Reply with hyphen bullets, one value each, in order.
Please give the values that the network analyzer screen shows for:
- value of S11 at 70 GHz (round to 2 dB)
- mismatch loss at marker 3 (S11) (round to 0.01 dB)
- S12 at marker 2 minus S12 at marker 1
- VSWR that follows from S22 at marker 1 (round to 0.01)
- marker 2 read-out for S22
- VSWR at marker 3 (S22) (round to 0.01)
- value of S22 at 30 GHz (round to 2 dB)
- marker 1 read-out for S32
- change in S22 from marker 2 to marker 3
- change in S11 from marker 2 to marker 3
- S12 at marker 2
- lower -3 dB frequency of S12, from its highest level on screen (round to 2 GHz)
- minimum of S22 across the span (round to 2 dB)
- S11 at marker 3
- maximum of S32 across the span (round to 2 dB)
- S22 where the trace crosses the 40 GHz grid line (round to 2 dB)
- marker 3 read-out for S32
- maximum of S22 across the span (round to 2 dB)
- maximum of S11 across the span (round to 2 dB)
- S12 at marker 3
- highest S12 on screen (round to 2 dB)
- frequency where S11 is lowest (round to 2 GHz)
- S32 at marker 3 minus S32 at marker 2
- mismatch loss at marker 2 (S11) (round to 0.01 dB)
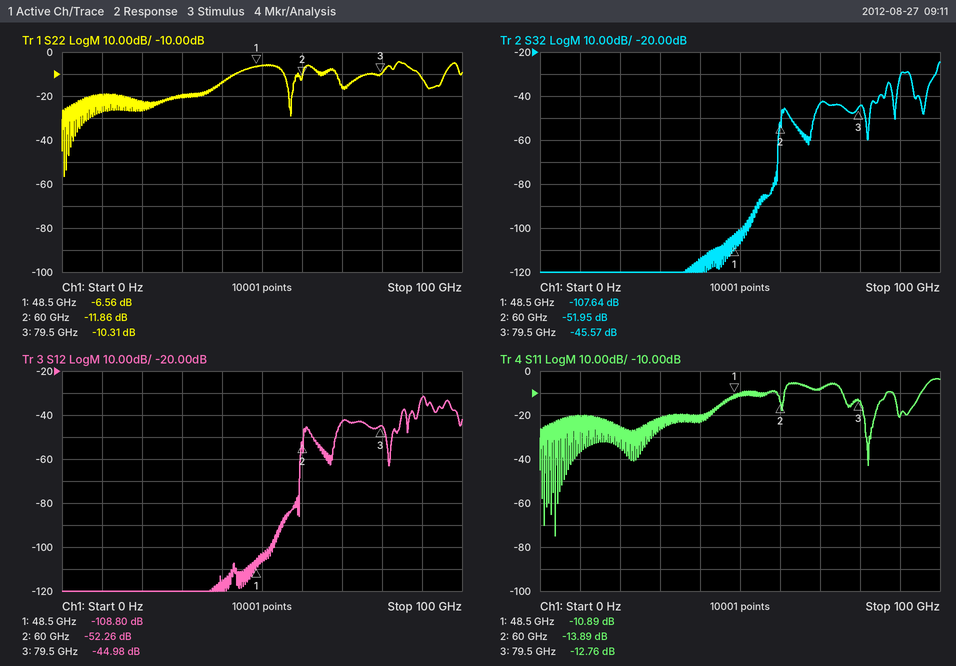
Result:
- -8 dB
- 0.24 dB
- 56.54 dB
- 2.77
- -11.86 dB
- 1.88
- -20 dB
- -107.64 dB
- 1.55 dB
- 1.13 dB
- -52.26 dB
- 90 GHz
- -56 dB
- -12.76 dB
- -24 dB
- -14 dB
- -45.57 dB
- -4 dB
- -4 dB
- -44.98 dB
- -32 dB
- 4 GHz
- 6.38 dB
- 0.18 dB
